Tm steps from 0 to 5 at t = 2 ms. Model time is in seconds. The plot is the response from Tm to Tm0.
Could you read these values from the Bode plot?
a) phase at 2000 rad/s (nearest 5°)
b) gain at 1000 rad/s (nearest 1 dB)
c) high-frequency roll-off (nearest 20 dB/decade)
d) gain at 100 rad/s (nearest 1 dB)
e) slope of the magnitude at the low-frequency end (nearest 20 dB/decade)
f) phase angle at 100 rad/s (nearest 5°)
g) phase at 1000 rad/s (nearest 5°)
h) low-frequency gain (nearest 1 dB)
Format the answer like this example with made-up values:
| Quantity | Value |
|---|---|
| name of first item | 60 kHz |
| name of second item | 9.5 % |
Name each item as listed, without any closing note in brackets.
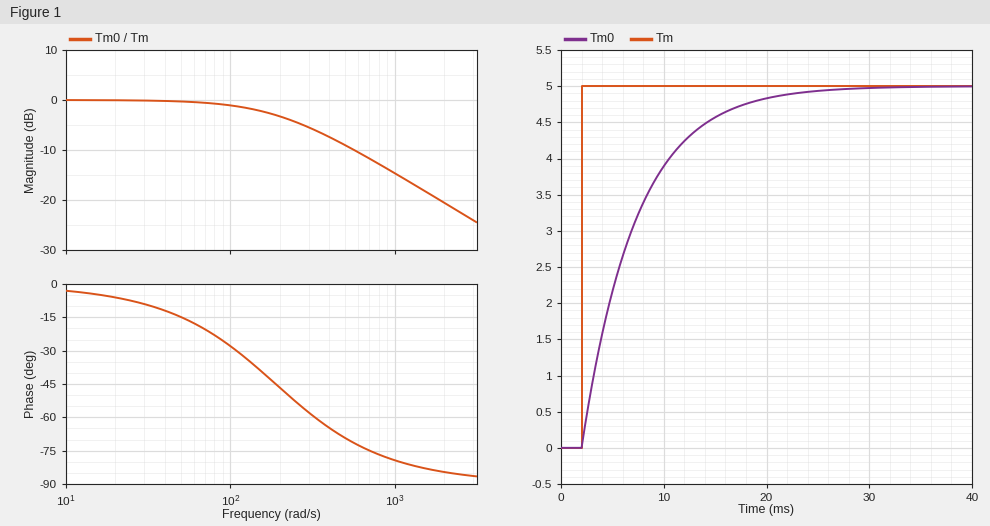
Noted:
| Quantity | Value |
|---|---|
| phase at 2000 rad/s | -85° |
| gain at 1000 rad/s | -15 dB |
| high-frequency roll-off | -20 dB/decade |
| gain at 100 rad/s | -1 dB |
| slope of the magnitude at the low-frequency end | 0 dB/decade |
| phase angle at 100 rad/s | -30° |
| phase at 1000 rad/s | -80° |
| low-frequency gain | 0 dB |
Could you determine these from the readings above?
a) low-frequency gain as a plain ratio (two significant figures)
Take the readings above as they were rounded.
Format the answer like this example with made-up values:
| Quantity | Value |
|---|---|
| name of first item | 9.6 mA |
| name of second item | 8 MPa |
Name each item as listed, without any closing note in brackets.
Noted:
| Quantity | Value |
|---|---|
| low-frequency gain as a plain ratio | 1.0 |
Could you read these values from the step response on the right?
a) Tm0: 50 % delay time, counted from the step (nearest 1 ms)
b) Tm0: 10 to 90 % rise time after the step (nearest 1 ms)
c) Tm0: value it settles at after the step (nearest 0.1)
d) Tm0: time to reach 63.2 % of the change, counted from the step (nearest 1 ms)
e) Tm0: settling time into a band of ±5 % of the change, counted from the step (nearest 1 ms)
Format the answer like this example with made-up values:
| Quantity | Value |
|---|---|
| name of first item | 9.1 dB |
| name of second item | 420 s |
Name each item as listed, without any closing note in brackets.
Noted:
| Quantity | Value |
|---|---|
| Tm0: 50 % delay time, counted from the step | 4 ms |
| Tm0: 10 to 90 % rise time after the step | 12 ms |
| Tm0: value it settles at after the step | 5.0 |
| Tm0: time to reach 63.2 % of the change, counted from the step | 5 ms |
| Tm0: settling time into a band of ±5 % of the change, counted from the step | 16 ms |
